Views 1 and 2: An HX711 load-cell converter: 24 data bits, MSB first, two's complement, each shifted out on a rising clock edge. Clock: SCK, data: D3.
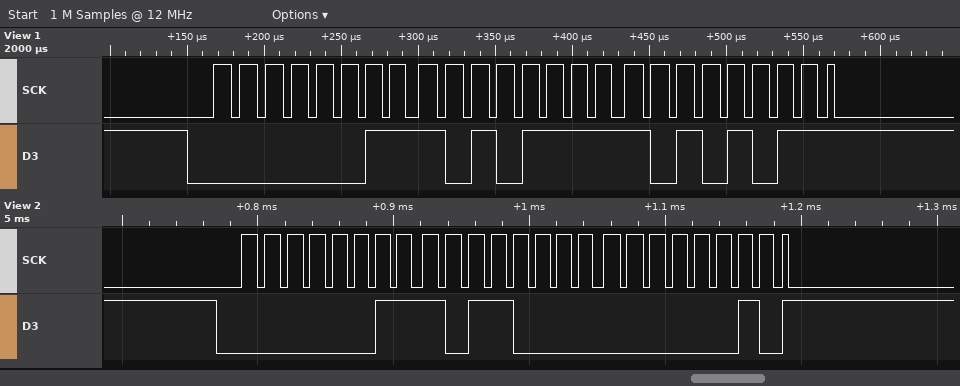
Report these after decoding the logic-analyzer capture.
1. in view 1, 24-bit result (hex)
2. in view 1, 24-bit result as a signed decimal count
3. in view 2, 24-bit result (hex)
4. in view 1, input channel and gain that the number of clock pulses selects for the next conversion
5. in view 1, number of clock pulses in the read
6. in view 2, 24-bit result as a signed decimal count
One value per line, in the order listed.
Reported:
0x03AFAB
241579
0x03B002
channel A, gain 128
25
241666
